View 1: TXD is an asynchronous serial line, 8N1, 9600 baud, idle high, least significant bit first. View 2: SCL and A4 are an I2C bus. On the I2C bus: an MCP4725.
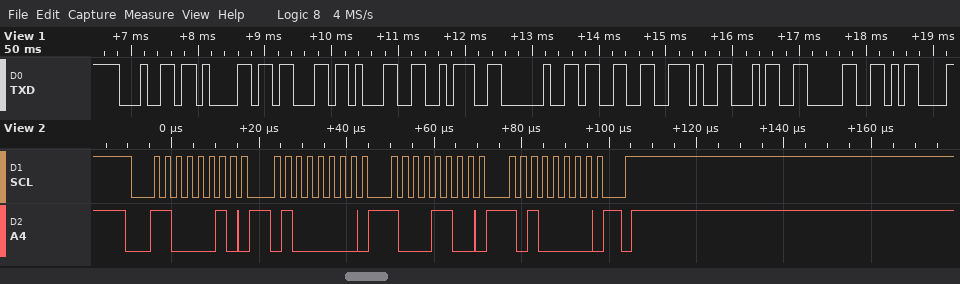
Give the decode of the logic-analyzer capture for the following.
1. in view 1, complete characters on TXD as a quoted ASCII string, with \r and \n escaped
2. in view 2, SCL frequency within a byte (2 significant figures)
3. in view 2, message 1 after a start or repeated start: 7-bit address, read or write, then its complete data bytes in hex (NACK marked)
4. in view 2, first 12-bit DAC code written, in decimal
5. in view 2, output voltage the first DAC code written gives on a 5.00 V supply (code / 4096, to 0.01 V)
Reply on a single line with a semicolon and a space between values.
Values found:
"dac1: 3.40\r"; 400 kHz; 0x61 write: 40 8C A0; 2250; 2.75 V
